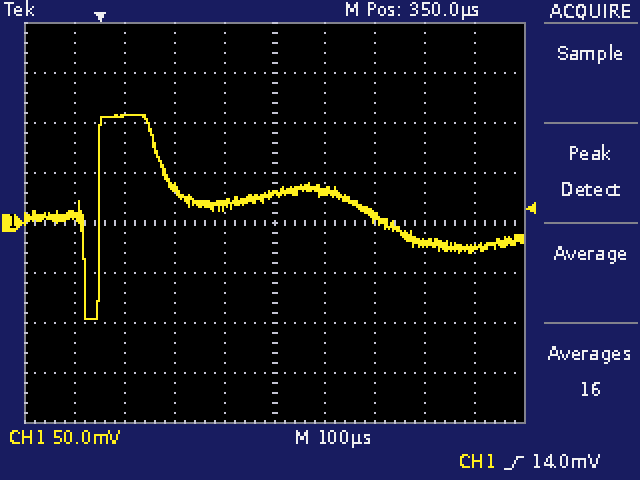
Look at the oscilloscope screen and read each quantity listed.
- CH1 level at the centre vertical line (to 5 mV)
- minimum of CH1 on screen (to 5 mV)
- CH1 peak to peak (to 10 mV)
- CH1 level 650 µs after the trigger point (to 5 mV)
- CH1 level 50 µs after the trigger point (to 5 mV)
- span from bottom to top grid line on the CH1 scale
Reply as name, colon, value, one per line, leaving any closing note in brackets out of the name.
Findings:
CH1 level at the centre vertical line: 30 mV
minimum of CH1 on screen: -95 mV
CH1 peak to peak: 200 mV
CH1 level 650 µs after the trigger point: -20 mV
CH1 level 50 µs after the trigger point: 105 mV
span from bottom to top grid line on the CH1 scale: 400 mV
